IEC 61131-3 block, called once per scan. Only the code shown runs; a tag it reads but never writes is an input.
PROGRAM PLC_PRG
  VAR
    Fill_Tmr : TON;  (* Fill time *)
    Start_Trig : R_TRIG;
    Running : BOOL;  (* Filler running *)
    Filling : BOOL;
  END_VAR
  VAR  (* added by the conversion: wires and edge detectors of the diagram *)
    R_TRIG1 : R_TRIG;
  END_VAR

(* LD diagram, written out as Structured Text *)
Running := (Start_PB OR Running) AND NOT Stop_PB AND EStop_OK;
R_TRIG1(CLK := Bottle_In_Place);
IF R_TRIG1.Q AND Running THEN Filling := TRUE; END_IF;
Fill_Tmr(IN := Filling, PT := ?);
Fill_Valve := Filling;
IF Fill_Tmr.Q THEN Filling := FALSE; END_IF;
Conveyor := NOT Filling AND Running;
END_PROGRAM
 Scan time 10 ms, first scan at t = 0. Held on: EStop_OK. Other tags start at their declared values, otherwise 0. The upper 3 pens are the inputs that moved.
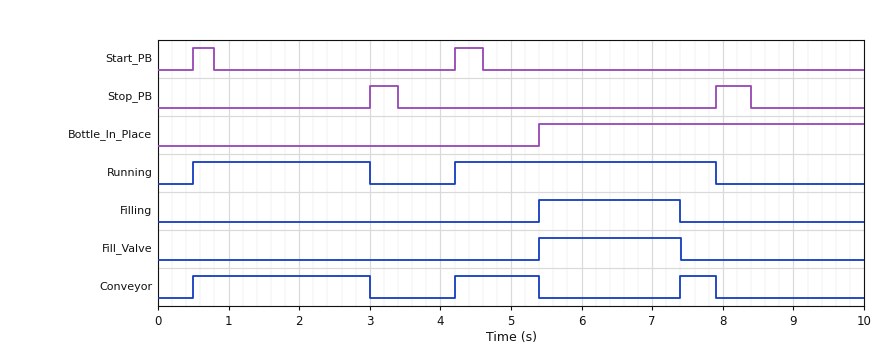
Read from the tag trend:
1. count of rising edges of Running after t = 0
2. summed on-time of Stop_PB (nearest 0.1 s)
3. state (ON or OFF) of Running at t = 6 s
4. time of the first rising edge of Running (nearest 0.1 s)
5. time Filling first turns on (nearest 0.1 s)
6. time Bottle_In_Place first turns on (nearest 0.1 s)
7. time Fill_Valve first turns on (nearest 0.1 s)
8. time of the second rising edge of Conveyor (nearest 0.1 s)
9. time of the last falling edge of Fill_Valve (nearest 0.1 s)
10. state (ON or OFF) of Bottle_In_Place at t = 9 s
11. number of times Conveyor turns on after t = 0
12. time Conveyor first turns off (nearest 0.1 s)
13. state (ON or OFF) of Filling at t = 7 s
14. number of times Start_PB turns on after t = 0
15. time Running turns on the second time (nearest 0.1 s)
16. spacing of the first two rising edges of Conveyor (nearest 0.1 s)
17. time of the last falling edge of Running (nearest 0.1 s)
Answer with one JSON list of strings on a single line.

["2", "0.9 s", "ON", "0.5 s", "5.4 s", "5.4 s", "5.4 s", "4.2 s", "7.4 s", "ON", "3", "3.0 s", "ON", "2", "4.2 s", "3.7 s", "7.9 s"]
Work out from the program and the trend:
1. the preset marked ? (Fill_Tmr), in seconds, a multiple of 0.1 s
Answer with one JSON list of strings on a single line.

["2.0 s"]
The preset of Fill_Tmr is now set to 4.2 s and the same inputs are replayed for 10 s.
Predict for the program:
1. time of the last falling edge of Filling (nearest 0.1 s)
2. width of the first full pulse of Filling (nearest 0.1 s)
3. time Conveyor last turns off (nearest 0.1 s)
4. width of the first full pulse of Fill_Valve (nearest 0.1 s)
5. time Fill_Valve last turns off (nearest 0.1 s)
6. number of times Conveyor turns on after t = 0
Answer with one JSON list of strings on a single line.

["9.6 s", "4.2 s", "5.4 s", "4.2 s", "9.6 s", "2"]
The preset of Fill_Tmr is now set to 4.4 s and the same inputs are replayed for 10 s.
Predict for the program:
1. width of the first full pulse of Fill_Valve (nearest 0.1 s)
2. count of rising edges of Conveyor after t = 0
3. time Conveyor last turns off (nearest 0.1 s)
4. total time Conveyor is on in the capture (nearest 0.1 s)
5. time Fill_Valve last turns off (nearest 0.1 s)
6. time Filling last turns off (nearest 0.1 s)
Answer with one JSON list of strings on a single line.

["4.4 s", "2", "5.4 s", "3.7 s", "9.8 s", "9.8 s"]
